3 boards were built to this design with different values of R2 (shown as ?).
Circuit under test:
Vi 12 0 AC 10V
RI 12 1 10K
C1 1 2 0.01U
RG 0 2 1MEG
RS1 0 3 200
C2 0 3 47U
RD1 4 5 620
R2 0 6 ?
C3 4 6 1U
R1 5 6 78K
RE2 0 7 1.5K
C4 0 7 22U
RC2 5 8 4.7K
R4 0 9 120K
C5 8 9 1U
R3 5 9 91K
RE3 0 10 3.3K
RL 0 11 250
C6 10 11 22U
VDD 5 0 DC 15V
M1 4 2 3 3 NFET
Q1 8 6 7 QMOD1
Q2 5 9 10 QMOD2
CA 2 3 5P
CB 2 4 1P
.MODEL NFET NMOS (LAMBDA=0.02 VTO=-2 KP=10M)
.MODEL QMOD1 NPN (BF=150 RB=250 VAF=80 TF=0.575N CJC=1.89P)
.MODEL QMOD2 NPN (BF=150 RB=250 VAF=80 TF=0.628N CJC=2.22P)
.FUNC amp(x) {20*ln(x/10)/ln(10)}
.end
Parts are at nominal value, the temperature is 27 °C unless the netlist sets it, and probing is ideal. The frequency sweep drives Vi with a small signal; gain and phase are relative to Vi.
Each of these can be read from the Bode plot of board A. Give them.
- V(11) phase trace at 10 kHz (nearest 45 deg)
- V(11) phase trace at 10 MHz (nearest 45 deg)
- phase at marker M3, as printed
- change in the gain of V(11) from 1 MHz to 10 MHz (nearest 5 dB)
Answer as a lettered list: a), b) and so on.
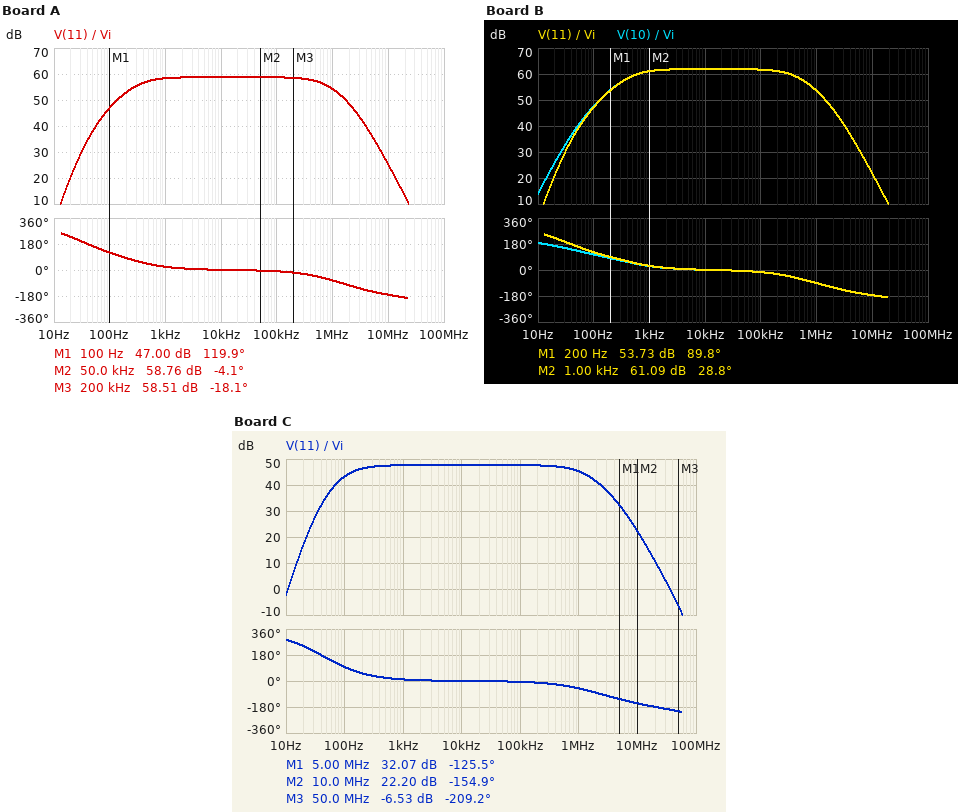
a) 0 deg
b) -180 deg
c) -18.1 deg
d) -30 dB
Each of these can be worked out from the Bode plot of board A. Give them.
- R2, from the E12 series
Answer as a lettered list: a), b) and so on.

a) 18 kΩ
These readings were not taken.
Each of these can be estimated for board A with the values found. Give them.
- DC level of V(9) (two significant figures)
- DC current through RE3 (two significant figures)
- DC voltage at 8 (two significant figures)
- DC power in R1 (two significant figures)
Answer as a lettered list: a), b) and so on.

a) 7.9 V
b) 2.1 mA
c) 9.0 V
d) 1.9 mW
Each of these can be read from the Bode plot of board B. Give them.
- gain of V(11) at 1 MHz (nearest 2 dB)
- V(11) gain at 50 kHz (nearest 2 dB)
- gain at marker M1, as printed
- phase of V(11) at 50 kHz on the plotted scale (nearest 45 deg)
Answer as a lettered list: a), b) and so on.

a) 54 dB
b) 62 dB
c) 53.73 dB
d) 0 deg
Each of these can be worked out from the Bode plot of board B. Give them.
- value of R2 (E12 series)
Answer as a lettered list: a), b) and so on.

a) 33 kΩ
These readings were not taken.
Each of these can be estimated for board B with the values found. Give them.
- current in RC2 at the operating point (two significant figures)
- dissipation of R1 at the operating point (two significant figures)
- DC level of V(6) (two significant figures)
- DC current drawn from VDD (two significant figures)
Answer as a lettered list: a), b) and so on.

a) 2.2 mA
b) 1.5 mW
c) 4.1 V
d) 9.9 mA
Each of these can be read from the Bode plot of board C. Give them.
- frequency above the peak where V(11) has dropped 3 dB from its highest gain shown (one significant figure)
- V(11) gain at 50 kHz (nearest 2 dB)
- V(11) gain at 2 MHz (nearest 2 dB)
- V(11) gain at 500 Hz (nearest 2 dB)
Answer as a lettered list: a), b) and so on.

a) 1 MHz
b) 48 dB
c) 42 dB
d) 48 dB
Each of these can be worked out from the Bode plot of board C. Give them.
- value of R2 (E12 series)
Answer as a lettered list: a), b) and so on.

a) 6.8 kΩ
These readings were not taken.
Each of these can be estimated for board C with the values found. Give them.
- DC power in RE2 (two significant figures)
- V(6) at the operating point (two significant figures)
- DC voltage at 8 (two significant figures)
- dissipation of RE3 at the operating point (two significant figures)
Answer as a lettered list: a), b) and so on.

a) 140 µW
b) 1.2 V
c) 14 V
d) 15 mW
